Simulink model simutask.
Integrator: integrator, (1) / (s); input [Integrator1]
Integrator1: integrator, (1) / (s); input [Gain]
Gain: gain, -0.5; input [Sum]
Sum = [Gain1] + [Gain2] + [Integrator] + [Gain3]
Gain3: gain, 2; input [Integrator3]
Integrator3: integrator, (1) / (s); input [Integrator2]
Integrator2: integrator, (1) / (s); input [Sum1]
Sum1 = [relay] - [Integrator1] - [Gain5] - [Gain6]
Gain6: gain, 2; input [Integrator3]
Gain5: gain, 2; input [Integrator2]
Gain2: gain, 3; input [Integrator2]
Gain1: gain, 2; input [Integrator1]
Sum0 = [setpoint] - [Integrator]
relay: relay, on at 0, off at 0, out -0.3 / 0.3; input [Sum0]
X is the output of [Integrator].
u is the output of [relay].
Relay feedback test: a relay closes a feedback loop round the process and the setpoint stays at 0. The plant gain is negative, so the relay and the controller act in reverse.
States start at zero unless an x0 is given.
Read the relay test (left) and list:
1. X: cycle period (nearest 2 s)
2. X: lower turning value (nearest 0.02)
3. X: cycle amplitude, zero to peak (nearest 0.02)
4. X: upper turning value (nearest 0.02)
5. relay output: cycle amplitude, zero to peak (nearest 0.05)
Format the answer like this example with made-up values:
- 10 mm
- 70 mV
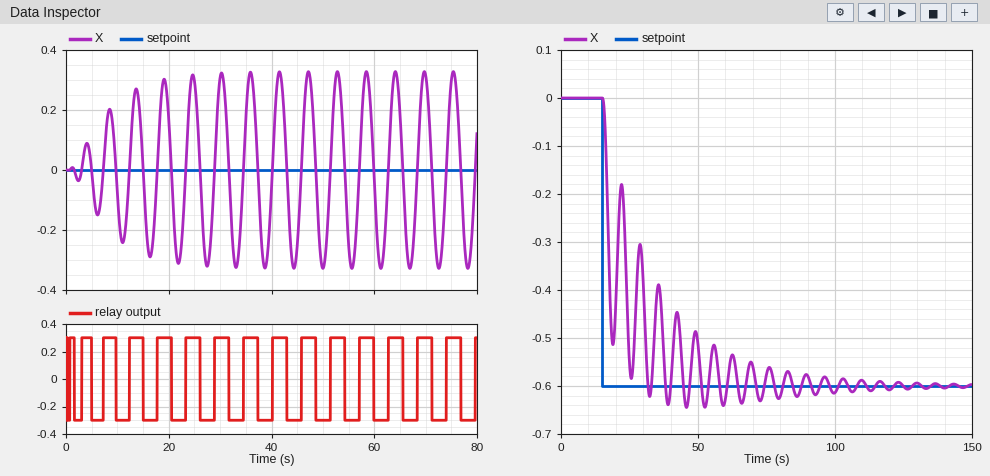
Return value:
- 6 s
- -0.32
- 0.32
- 0.32
- 0.30
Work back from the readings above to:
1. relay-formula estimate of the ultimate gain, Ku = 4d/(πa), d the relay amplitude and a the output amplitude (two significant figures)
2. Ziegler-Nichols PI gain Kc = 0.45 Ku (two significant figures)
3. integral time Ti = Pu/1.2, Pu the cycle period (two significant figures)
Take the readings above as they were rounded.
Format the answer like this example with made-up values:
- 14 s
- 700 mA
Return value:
- 1.2
- 0.54
- 5.0 s
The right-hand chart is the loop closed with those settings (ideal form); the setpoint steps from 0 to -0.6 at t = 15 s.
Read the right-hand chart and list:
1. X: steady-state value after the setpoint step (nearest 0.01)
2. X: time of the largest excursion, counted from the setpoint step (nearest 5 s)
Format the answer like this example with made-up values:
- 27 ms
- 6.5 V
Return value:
- -0.60
- 30 s
